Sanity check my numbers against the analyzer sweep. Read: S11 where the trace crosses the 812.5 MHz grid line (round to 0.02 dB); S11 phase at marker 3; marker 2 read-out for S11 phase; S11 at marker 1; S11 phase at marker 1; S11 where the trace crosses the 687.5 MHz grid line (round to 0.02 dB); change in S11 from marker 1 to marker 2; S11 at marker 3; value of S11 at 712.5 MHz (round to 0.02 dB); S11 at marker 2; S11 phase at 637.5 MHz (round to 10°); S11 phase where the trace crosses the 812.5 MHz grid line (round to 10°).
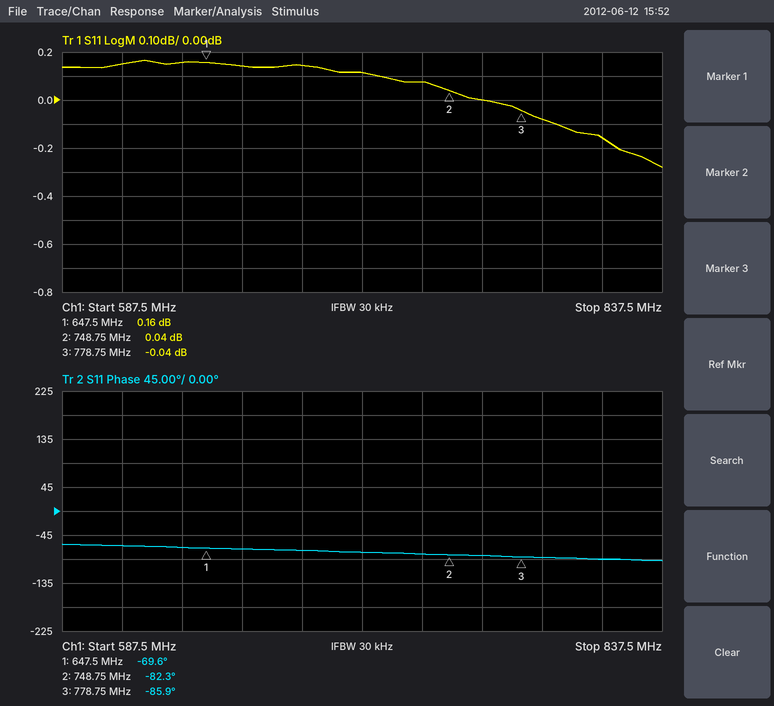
-0.16 dB
-85.9°
-82.3°
0.16 dB
-69.6°
0.14 dB
-0.12 dB
-0.04 dB
0.12 dB
0.04 dB
-70°
-90°
